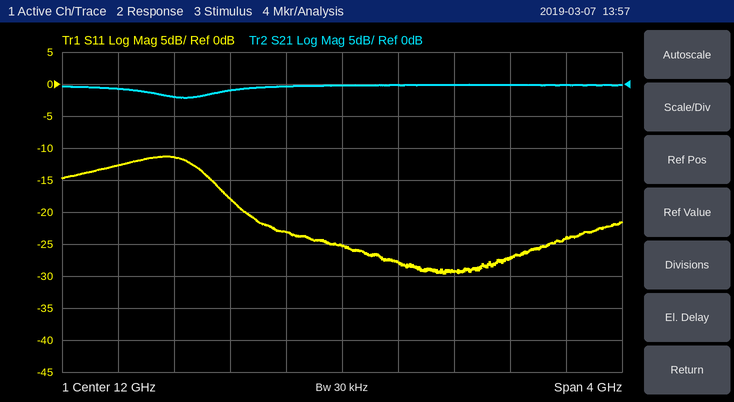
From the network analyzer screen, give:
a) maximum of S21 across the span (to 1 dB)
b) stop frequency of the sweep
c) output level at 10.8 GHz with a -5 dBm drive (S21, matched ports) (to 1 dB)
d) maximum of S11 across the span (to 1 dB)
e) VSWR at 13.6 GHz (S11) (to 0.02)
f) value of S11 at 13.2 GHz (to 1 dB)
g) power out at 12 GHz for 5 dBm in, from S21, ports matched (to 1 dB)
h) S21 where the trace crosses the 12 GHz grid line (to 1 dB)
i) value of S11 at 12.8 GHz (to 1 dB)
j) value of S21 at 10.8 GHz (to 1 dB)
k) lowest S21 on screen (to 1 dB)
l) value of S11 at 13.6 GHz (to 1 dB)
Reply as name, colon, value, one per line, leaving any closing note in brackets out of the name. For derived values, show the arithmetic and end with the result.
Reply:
maximum of S21 across the span: 0 dB
stop frequency of the sweep: 14 GHz
output level at 10.8 GHz with a -5 dBm drive (S21, matched ports): -5 dBm + (-2 dB) = -7 dBm
maximum of S11 across the span: -11 dB
VSWR at 13.6 GHz (S11): |Γ| = 10^(-24/20) = 0.0631; VSWR = (1 + 0.0631)/(1 − 0.0631) ≈ 1.13, so 1.14 to the nearest 0.02
value of S11 at 13.2 GHz: -27 dB
power out at 12 GHz for 5 dBm in, from S21, ports matched: 5 dBm + (0 dB) = 5 dBm
S21 where the trace crosses the 12 GHz grid line: 0 dB
value of S11 at 12.8 GHz: -29 dB
value of S21 at 10.8 GHz: -2 dB
lowest S21 on screen: -2 dB
value of S11 at 13.6 GHz: -24 dB
